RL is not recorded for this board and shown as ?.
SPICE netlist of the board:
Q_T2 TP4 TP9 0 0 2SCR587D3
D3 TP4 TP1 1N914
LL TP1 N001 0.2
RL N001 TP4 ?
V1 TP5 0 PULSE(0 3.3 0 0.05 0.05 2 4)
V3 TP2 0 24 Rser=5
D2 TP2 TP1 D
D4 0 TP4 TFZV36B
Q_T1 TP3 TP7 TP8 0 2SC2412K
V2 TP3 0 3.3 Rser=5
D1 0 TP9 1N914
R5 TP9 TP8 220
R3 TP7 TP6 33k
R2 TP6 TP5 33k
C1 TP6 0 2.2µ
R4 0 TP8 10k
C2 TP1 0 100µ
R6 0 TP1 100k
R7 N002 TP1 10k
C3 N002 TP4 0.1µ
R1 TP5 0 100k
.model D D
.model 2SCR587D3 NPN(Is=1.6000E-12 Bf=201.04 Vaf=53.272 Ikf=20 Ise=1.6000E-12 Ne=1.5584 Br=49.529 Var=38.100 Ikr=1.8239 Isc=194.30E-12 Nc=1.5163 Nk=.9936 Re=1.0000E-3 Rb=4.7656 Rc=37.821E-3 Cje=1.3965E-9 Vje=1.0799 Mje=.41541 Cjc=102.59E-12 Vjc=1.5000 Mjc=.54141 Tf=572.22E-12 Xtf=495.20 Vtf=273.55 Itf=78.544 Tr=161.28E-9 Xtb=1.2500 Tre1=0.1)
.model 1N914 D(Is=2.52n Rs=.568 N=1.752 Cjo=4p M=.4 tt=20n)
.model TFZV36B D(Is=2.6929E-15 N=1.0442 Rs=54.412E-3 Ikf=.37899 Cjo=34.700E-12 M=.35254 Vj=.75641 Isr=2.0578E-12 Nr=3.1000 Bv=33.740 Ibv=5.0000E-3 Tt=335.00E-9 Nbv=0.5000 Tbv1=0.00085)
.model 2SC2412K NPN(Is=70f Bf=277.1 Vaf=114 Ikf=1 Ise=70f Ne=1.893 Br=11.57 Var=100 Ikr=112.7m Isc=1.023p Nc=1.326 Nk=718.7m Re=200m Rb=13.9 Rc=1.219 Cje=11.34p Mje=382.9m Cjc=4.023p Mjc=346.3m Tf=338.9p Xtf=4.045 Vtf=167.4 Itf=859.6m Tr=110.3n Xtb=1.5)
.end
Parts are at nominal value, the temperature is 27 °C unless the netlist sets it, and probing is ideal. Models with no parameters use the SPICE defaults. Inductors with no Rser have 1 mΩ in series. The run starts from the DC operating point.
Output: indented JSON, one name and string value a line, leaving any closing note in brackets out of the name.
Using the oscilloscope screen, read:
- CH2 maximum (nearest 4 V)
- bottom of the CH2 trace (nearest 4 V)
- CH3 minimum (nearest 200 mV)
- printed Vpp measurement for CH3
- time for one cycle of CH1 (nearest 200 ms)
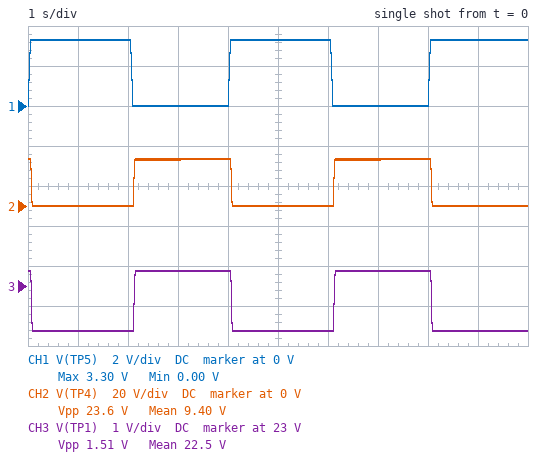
{
  "CH2 maximum": "24 V",
  "bottom of the CH2 trace": "0 V",
  "CH3 minimum": "21.8 V",
  "printed Vpp measurement for CH3": "1.51 V",
  "time for one cycle of CH1": "4.0 s"
}
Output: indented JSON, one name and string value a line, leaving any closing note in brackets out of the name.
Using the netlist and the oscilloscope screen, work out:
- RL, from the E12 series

{
  "RL, from the E12 series": "82 Ω"
}
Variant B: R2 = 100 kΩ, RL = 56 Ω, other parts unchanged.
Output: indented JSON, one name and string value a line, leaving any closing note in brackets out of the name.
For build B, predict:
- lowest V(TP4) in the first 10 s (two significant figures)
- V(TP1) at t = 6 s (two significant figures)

{
  "lowest V(TP4) in the first 10 s": "120 mV",
  "V(TP1) at t = 6 s": "21 V"
}
